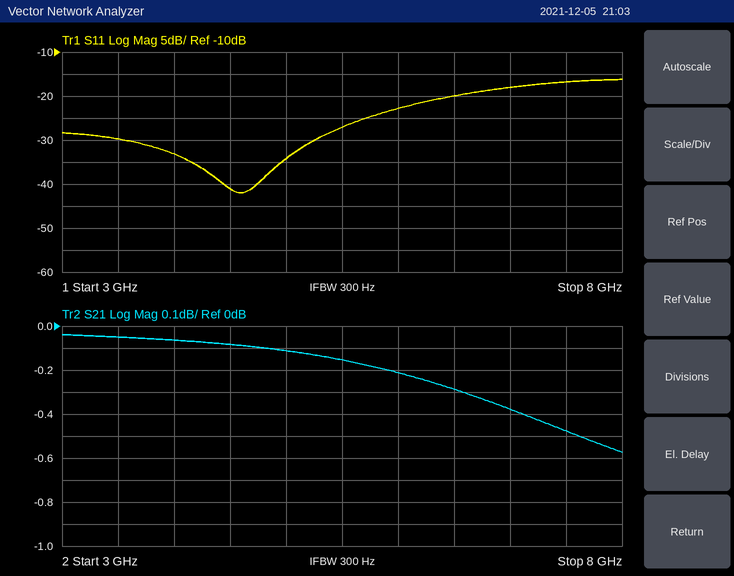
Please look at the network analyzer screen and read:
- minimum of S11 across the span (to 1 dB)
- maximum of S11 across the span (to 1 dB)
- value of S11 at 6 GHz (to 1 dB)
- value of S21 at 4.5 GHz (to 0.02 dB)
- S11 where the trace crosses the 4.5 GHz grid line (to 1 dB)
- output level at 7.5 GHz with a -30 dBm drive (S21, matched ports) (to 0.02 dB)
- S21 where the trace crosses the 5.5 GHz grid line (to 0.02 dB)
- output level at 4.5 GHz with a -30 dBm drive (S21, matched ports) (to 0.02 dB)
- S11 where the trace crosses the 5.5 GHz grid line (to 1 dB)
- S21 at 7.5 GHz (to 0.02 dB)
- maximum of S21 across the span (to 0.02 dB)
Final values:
-42 dB
-16 dB
-23 dB
-0.08 dB
-41 dB
-30.48 dBm
-0.16 dB
-30.08 dBm
-27 dB
-0.48 dB
-0.04 dB
